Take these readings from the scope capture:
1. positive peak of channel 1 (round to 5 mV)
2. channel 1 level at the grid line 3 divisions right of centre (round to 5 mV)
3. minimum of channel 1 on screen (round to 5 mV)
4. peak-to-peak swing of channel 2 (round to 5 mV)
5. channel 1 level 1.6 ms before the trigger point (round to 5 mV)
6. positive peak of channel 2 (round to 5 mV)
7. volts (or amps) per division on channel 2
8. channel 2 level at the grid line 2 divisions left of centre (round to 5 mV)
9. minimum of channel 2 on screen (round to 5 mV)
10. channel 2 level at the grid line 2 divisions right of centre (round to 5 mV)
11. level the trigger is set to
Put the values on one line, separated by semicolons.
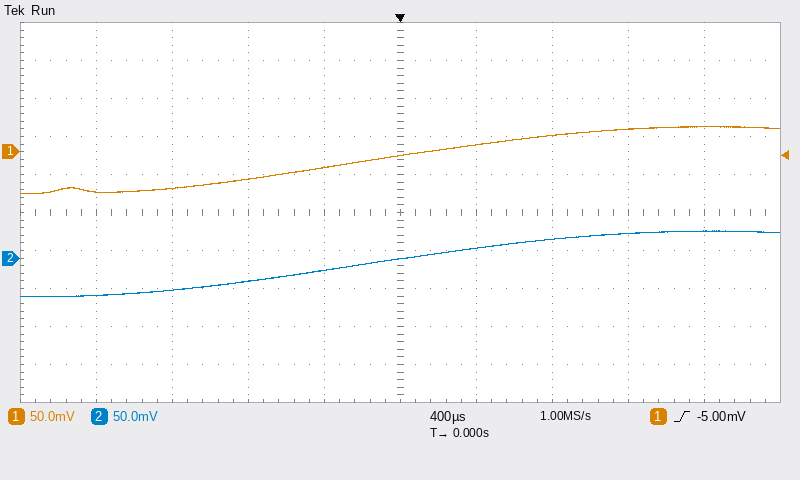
35 mV; 30 mV; -55 mV; 85 mV; -55 mV; 35 mV; 50 mV; -30 mV; -50 mV; 25 mV; -5.00 mV
